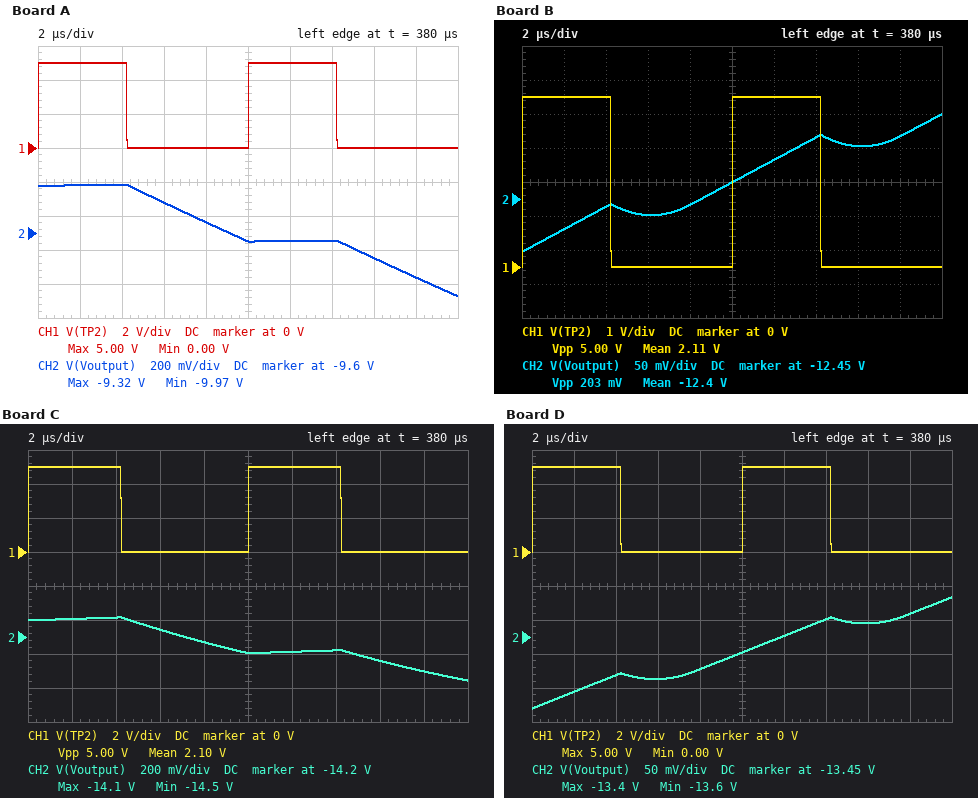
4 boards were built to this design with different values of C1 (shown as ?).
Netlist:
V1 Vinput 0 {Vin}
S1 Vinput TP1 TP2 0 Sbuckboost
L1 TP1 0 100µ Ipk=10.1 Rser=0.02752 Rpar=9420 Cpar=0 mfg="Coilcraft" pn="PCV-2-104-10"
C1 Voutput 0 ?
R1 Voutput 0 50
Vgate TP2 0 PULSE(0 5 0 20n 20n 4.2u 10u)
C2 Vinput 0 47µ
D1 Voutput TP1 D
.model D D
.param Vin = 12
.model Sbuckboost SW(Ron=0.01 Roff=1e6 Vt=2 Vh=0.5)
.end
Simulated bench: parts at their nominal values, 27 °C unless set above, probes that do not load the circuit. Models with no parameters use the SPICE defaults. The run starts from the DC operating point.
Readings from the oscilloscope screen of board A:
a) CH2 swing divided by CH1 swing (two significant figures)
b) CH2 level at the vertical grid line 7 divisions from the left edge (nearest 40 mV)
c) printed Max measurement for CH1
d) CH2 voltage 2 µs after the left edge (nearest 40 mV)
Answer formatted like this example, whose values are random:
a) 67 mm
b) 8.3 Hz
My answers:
a) 0.13
b) -9.64 V
c) 5.00 V
d) -9.32 V
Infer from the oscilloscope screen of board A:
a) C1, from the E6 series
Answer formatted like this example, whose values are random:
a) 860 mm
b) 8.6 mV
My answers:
a) 150 µF
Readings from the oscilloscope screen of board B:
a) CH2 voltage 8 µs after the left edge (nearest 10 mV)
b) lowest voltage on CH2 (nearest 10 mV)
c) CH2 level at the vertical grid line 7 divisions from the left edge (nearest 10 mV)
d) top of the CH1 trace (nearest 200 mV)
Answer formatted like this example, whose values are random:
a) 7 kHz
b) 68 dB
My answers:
a) -12.46 V
b) -12.53 V
c) -12.36 V
d) 5.0 V
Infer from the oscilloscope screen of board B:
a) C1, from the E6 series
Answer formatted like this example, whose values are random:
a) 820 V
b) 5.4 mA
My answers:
a) 15 µF
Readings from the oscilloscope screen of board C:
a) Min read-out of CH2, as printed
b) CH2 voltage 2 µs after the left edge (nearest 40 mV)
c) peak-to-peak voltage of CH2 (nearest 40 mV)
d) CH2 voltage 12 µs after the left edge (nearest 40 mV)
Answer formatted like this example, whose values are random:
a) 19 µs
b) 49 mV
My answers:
a) -14.5 V
b) -14.08 V
c) 360 mV
d) -14.28 V
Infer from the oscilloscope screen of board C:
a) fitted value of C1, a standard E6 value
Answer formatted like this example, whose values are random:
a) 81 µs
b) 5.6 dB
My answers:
a) 68 µF
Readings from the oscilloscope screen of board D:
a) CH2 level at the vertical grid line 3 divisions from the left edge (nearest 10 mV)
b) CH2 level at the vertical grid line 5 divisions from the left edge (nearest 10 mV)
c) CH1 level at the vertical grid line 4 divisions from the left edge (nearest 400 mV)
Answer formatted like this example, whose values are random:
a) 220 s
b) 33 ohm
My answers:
a) -13.51 V
b) -13.47 V
c) 0 V
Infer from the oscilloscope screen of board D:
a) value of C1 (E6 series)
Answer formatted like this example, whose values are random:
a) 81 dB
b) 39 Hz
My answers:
a) 22 µF
